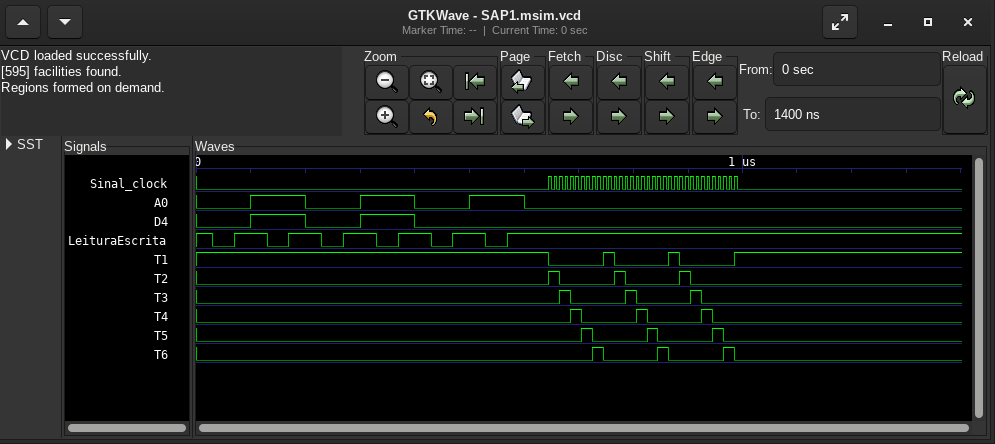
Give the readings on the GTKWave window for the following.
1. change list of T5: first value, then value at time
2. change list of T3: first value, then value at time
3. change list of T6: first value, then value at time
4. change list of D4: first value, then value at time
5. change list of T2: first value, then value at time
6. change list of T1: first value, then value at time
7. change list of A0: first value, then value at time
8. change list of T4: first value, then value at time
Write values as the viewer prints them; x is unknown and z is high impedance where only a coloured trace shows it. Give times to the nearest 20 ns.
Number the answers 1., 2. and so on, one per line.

1. 0, 1 at 700 ns, 0 at 720 ns, 1 at 820 ns, 0 at 840 ns, 1 at 940 ns, 0 at 960 ns
2. 0, 1 at 660 ns, 0 at 680 ns, 1 at 780 ns, 0 at 800 ns, 1 at 900 ns, 0 at 920 ns
3. 0, 1 at 720 ns, 0 at 740 ns, 1 at 840 ns, 0 at 860 ns, 1 at 960 ns, 0 at 980 ns
4. 0, 1 at 100 ns, 0 at 200 ns, 1 at 300 ns, 0 at 400 ns
5. 0, 1 at 640 ns, 0 at 660 ns, 1 at 760 ns, 0 at 780 ns, 1 at 880 ns, 0 at 900 ns
6. 1, 0 at 640 ns, 1 at 740 ns, 0 at 760 ns, 1 at 860 ns, 0 at 880 ns, 1 at 980 ns
7. 0, 1 at 100 ns, 0 at 200 ns, 1 at 300 ns, 0 at 400 ns, 1 at 500 ns, 0 at 600 ns
8. 0, 1 at 680 ns, 0 at 700 ns, 1 at 800 ns, 0 at 820 ns, 1 at 920 ns, 0 at 940 ns
